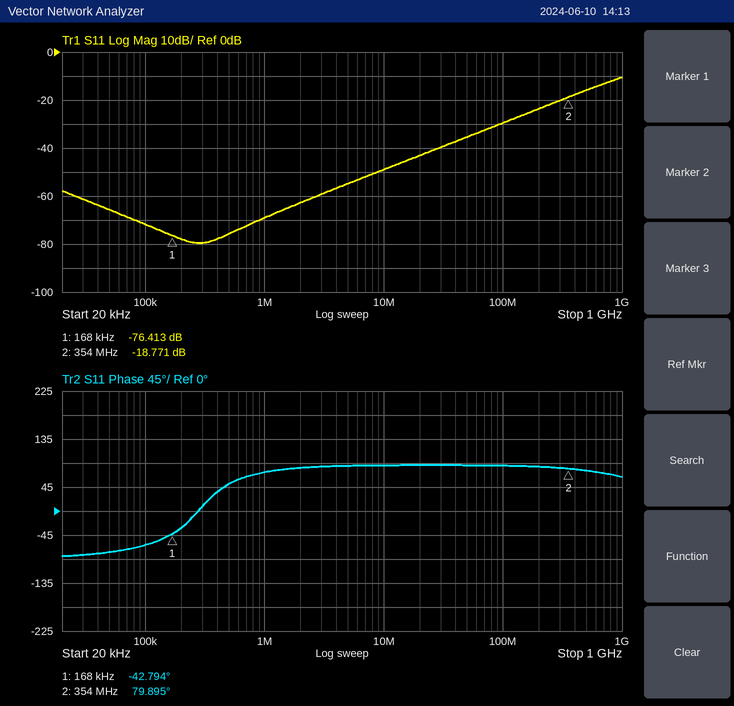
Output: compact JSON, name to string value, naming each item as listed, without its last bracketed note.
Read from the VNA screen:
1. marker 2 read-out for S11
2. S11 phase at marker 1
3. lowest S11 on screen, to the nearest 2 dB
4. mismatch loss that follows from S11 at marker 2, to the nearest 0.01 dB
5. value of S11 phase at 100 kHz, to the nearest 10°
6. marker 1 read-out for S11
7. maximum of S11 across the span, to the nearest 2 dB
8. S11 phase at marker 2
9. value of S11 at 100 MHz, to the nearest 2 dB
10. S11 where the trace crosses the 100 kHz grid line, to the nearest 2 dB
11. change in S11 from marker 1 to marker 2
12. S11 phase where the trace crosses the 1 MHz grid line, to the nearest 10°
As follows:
{"marker 2 read-out for S11": "-18.771 dB", "S11 phase at marker 1": "-42.794°", "lowest S11 on screen, to the nearest 2 dB": "-80 dB", "mismatch loss that follows from S11 at marker 2, to the nearest 0.01 dB": "0.06 dB", "value of S11 phase at 100 kHz, to the nearest 10°": "-60°", "marker 1 read-out for S11": "-76.413 dB", "maximum of S11 across the span, to the nearest 2 dB": "-10 dB", "S11 phase at marker 2": "79.895°", "value of S11 at 100 MHz, to the nearest 2 dB": "-30 dB", "S11 where the trace crosses the 100 kHz grid line, to the nearest 2 dB": "-72 dB", "change in S11 from marker 1 to marker 2": "57.642 dB", "S11 phase where the trace crosses the 1 MHz grid line, to the nearest 10°": "70°"}
